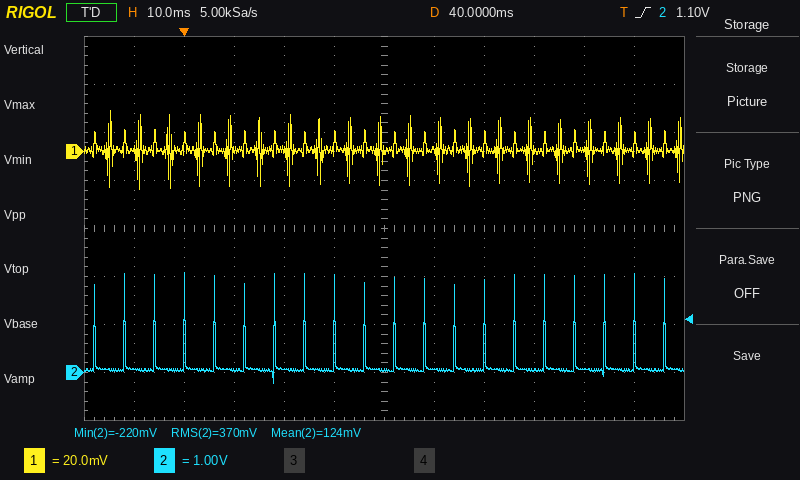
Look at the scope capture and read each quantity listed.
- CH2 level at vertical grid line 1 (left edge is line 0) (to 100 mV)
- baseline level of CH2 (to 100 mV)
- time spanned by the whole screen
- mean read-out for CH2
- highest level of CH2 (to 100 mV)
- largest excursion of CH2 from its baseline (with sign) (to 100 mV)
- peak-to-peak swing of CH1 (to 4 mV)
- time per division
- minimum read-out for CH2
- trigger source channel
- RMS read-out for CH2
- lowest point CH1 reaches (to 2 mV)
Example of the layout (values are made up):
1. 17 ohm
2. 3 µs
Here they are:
1. 100 mV
2. 100 mV
3. 120 ms
4. 124 mV
5. 2.1 V
6. +2.0 V
7. 32 mV
8. 10 ms
9. -220 mV
10. CH2
11. 370 mV
12. -16 mV
